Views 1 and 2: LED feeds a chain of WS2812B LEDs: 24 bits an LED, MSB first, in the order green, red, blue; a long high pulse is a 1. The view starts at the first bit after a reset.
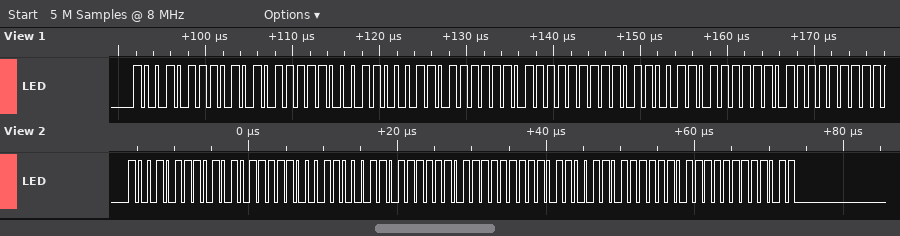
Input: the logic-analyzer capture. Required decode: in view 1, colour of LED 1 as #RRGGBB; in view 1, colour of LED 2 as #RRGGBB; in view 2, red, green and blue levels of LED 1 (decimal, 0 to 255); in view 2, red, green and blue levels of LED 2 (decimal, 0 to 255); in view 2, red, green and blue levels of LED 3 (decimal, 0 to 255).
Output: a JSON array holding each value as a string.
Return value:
["#5797C6", "#EF37FB", "87, 151, 198", "239, 55, 251", "239, 55, 251"]
